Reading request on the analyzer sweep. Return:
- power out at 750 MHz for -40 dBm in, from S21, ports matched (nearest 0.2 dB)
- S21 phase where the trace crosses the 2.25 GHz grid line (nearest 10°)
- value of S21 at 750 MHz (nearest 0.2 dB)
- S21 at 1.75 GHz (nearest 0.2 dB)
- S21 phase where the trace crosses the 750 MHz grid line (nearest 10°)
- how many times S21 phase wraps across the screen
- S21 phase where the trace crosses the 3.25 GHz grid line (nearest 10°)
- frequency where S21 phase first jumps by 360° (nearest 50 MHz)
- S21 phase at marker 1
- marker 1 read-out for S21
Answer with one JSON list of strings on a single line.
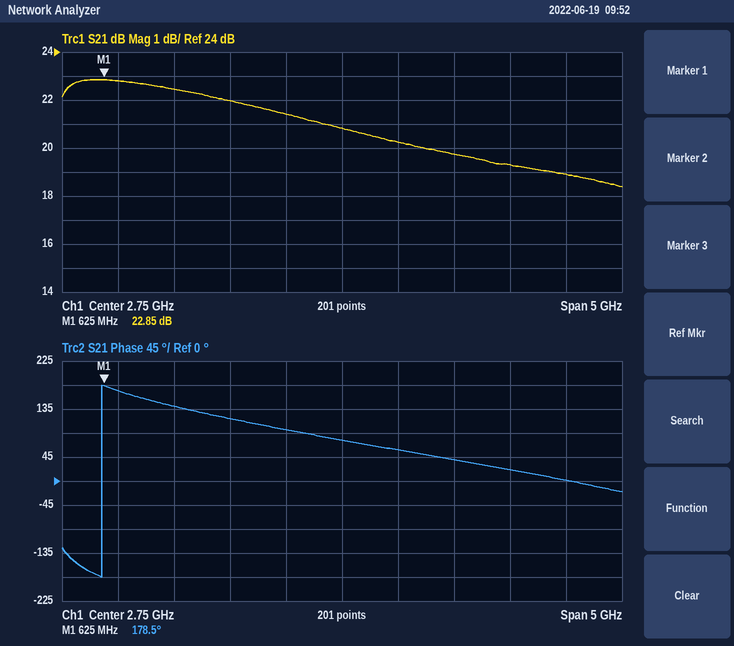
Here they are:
["-17.2 dBm", "100°", "22.8 dB", "22.0 dB", "170°", "1", "60°", "600 MHz", "178.5°", "22.85 dB"]
